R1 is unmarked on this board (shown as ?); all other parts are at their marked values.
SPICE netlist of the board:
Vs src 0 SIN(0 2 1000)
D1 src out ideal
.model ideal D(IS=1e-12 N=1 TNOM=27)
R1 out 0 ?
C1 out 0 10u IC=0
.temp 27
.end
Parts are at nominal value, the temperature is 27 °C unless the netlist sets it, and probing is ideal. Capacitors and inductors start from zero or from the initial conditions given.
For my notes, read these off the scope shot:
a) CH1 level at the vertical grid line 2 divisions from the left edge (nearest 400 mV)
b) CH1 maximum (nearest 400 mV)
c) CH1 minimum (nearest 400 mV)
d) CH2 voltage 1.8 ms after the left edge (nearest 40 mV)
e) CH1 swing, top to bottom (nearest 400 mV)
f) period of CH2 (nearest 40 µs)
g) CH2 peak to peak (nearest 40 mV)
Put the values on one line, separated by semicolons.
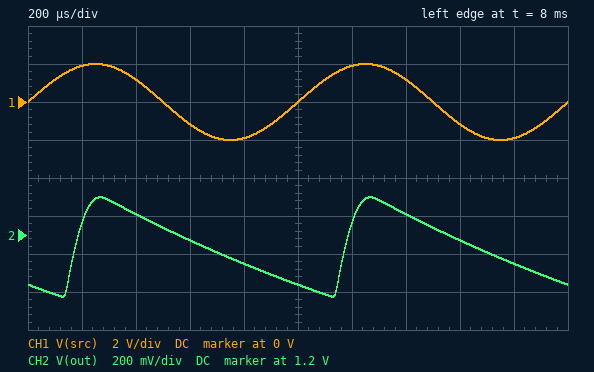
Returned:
1.2 V; 2.0 V; -2.0 V; 1.04 V; 4.0 V; 1.00 ms; 520 mV
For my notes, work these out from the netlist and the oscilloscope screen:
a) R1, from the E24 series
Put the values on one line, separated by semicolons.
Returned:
180 Ω
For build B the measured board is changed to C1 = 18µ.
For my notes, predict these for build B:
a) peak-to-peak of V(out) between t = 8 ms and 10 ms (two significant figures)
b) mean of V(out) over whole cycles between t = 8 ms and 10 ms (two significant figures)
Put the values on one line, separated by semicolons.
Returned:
330 mV; 1.2 V
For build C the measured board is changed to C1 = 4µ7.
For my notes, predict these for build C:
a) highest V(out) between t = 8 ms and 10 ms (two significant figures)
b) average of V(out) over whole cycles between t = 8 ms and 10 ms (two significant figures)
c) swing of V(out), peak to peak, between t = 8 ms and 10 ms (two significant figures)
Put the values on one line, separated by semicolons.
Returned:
1.4 V; 940 mV; 870 mV
